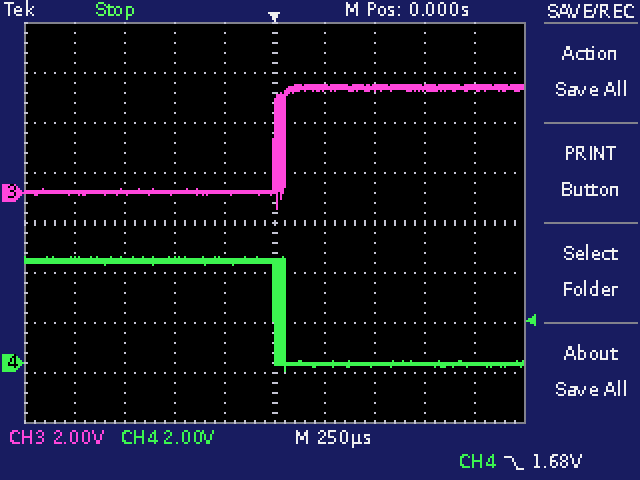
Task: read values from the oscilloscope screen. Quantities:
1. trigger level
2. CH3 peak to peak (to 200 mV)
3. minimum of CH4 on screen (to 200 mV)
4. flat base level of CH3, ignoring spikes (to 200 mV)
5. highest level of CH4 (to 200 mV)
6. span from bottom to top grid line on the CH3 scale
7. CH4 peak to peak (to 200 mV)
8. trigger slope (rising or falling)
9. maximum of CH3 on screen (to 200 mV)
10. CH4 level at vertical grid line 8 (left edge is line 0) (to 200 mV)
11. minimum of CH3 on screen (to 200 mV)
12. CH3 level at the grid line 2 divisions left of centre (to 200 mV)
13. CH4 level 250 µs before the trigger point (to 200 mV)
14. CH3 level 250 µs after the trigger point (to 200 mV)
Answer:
1.68 V
5.0 V
-400 mV
0.0 V
4.2 V
16 V
4.6 V
falling
4.4 V
0.0 V
-600 mV
0.0 V
4.0 V
4.2 V
